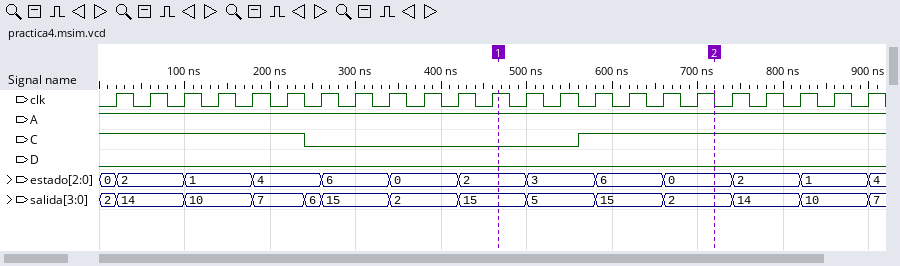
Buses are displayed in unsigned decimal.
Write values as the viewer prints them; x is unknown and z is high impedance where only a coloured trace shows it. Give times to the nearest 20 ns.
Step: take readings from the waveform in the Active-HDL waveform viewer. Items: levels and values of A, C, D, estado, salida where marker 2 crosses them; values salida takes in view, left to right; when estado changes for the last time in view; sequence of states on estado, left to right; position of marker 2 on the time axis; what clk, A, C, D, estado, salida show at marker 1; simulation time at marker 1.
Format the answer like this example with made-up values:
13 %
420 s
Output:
A=1, C=1, D=0, estado=0, salida=2
2, 14, 10, 7, 6, 15, 2, 15, 5, 15, 2, 14, 10, 7
900 ns
0, 2, 1, 4, 6, 0, 2, 3, 6, 0, 2, 1, 4
720 ns
clk=1, A=1, C=0, D=0, estado=2, salida=15
460 ns
